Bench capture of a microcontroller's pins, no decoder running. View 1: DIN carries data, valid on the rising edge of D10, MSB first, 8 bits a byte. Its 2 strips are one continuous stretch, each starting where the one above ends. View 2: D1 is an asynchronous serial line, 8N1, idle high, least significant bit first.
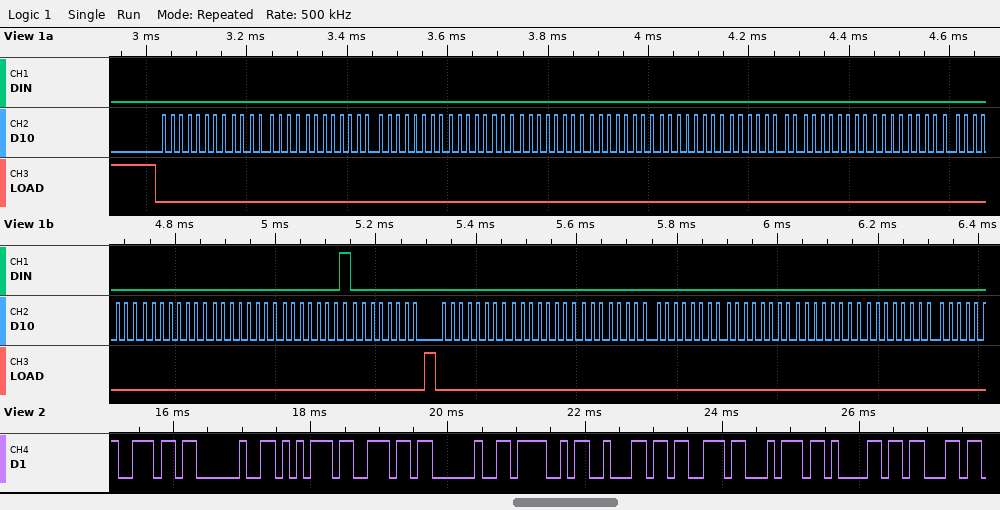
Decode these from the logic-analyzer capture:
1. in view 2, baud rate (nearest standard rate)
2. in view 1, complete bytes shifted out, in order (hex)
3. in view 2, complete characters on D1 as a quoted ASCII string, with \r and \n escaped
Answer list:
9600 baud
0x00 0x00 0x00 0x00 0x00 0x00 0x00 0x00 0x00 0x00 0x00 0x00 0x00 0x00 0x01 0x00 0x00 0x00 0x00 0x00 0x00 0x00 0x00
"n un Obstac"
